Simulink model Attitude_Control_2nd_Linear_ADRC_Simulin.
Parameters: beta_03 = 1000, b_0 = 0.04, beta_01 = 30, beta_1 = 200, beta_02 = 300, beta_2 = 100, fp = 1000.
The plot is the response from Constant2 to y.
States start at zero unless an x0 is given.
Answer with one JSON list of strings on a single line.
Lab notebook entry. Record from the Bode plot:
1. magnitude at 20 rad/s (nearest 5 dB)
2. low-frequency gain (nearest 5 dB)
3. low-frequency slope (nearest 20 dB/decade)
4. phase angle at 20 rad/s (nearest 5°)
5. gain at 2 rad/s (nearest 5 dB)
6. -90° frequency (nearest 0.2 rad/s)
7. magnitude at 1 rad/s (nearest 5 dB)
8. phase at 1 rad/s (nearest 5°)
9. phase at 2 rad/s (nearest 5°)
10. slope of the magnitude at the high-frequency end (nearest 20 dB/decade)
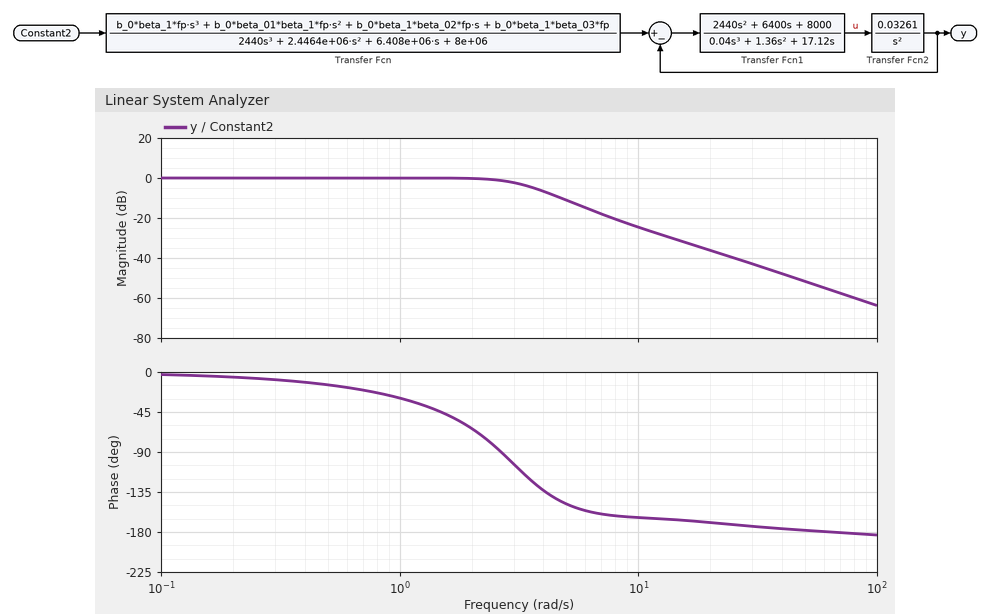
["-35 dB", "0 dB", "0 dB/decade", "-170°", "0 dB", "2.6 rad/s", "0 dB", "-30°", "-65°", "-40 dB/decade"]
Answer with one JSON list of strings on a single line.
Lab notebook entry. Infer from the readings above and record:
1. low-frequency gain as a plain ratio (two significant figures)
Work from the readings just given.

["1.0"]
